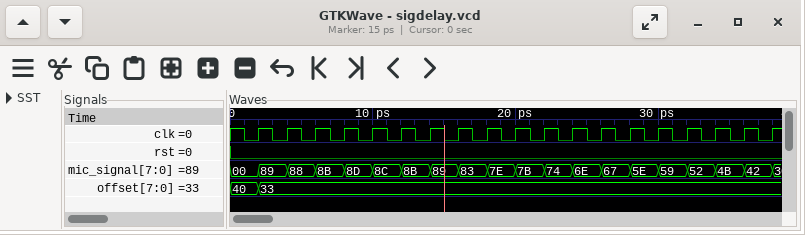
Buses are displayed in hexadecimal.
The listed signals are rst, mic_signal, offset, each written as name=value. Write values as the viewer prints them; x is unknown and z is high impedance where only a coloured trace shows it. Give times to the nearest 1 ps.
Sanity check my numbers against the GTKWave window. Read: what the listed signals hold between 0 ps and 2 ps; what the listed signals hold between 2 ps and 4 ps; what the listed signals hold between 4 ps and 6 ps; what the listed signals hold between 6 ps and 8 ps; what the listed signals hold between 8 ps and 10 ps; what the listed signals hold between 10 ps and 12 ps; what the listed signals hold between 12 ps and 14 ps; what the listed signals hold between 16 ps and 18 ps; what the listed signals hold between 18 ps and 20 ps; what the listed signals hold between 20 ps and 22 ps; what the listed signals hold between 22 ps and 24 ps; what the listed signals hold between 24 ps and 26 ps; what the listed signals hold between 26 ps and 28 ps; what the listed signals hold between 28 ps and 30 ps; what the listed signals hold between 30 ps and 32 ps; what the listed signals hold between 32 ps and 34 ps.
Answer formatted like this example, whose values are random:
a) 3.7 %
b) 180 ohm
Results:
a) rst=0, mic_signal=00, offset=40
b) rst=0, mic_signal=89, offset=33
c) rst=0, mic_signal=88, offset=33
d) rst=0, mic_signal=8B, offset=33
e) rst=0, mic_signal=8D, offset=33
f) rst=0, mic_signal=8C, offset=33
g) rst=0, mic_signal=8B, offset=33
h) rst=0, mic_signal=83, offset=33
i) rst=0, mic_signal=7E, offset=33
j) rst=0, mic_signal=7B, offset=33
k) rst=0, mic_signal=74, offset=33
l) rst=0, mic_signal=6E, offset=33
m) rst=0, mic_signal=67, offset=33
n) rst=0, mic_signal=5E, offset=33
o) rst=0, mic_signal=59, offset=33
p) rst=0, mic_signal=52, offset=33
